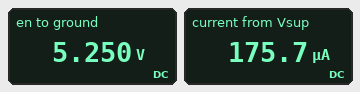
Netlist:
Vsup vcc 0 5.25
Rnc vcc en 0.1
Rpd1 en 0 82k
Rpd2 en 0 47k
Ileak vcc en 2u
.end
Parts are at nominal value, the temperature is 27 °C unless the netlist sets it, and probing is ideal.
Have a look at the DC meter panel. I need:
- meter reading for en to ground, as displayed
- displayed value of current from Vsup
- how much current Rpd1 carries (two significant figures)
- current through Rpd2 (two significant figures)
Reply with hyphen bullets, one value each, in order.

- 5.250 V
- 175.7 µA
- 64 µA
- 110 µA
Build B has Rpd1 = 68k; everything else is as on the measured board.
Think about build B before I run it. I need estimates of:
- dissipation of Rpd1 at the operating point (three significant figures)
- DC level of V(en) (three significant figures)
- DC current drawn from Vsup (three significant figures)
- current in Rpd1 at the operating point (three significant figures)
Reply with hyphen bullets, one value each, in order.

- 405 µW
- 5.25 V
- 189 µA
- 77.2 µA
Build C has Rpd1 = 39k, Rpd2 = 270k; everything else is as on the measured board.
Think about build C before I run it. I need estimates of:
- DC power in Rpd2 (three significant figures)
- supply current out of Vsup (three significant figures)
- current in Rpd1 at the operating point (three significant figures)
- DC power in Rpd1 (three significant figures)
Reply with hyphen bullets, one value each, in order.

- 102 µW
- 154 µA
- 135 µA
- 707 µW
